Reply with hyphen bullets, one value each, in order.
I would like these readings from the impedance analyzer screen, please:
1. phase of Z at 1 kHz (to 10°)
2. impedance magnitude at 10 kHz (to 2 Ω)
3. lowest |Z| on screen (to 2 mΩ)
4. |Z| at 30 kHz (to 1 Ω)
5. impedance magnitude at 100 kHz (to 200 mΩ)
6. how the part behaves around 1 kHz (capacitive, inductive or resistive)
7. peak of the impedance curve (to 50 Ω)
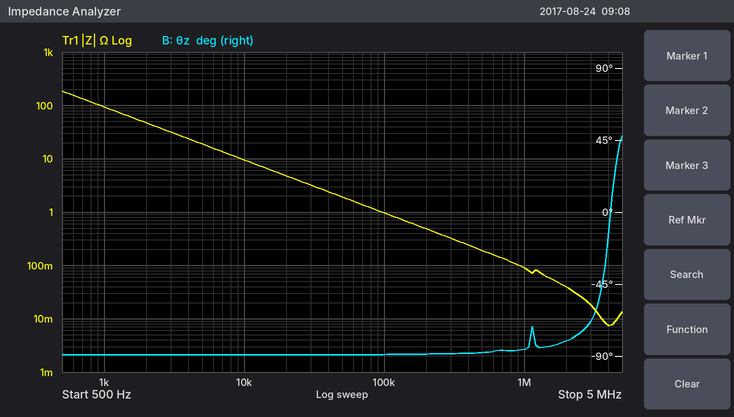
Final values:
- -90°
- 10 Ω
- 8 mΩ
- 3 Ω
- 1.0 Ω
- capacitive
- 200 Ω
